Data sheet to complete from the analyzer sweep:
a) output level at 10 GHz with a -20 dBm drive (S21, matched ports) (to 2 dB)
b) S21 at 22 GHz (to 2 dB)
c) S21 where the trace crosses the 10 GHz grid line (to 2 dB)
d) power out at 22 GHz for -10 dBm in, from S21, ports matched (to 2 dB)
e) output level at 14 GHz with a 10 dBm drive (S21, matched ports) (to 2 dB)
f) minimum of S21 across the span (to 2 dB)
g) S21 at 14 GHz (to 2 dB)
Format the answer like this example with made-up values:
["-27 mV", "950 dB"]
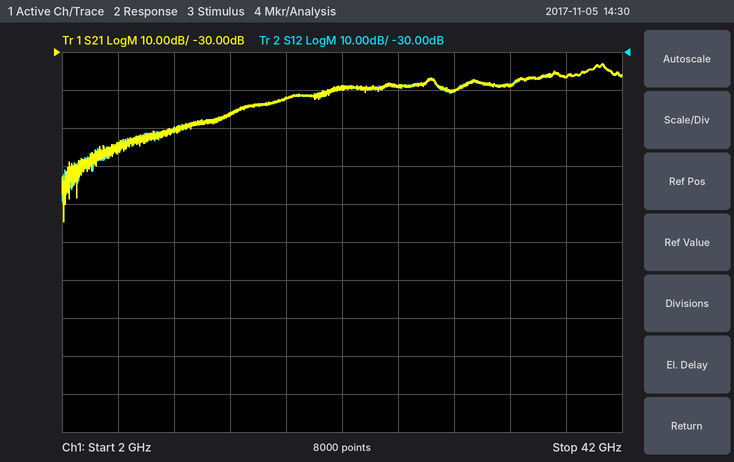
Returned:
["-70 dBm", "-40 dB", "-50 dB", "-50 dBm", "-36 dBm", "-74 dB", "-46 dB"]
